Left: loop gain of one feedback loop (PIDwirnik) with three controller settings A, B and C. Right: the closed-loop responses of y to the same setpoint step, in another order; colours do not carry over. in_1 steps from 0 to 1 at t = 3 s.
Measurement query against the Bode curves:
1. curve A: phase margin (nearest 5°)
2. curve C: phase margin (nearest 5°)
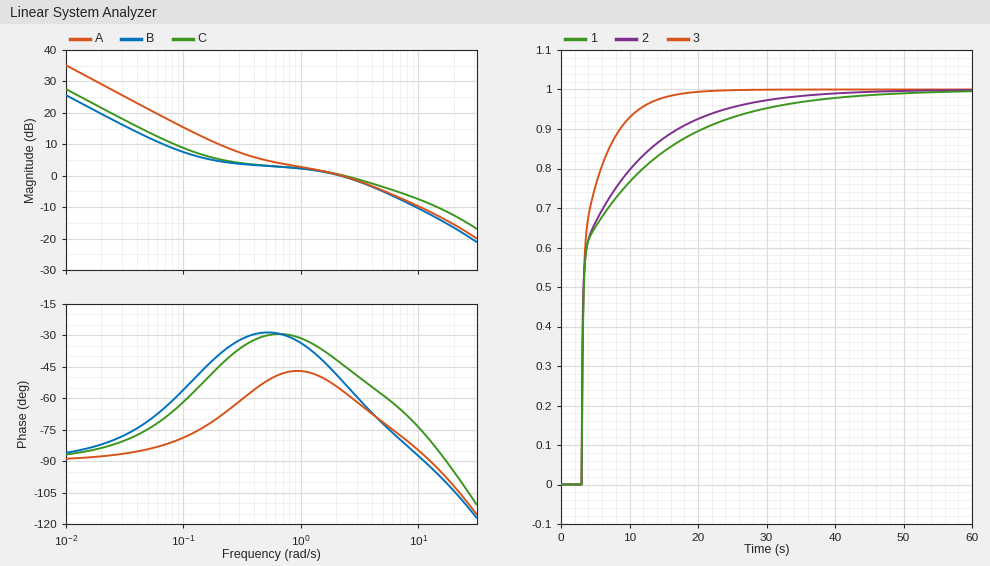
125°
135°
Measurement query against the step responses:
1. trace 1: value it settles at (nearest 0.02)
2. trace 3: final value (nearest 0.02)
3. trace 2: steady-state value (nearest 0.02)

1.00
1.00
1.00
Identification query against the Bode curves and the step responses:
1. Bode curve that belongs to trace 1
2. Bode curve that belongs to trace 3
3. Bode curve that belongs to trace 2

B
A
C
